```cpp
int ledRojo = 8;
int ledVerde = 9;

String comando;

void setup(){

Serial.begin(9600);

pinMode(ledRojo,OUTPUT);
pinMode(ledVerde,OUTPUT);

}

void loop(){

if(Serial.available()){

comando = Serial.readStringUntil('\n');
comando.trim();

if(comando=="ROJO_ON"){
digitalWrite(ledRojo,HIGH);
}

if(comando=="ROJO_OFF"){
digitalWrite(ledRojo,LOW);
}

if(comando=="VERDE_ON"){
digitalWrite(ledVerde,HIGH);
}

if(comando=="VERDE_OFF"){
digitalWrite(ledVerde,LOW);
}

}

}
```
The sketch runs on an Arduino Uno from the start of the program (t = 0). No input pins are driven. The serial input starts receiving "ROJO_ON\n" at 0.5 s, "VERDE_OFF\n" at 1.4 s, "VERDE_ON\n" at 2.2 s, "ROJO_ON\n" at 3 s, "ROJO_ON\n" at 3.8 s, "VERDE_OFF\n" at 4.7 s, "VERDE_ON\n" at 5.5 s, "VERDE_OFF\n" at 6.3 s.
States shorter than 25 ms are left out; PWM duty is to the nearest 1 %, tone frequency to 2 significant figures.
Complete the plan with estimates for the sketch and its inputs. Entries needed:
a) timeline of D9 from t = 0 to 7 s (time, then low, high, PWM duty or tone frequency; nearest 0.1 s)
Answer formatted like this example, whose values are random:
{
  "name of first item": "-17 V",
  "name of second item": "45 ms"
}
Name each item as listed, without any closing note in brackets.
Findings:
{
  "timeline of D9 from t = 0 to 7 s": "0 s low; 2.2 s high; 4.7 s low; 5.5 s high; 6.3 s low"
}
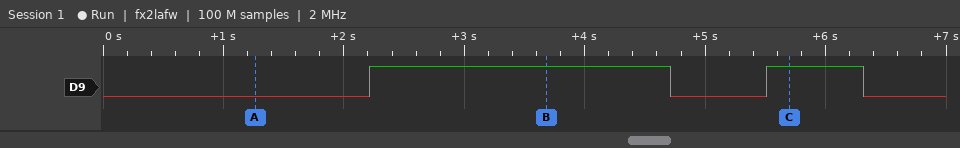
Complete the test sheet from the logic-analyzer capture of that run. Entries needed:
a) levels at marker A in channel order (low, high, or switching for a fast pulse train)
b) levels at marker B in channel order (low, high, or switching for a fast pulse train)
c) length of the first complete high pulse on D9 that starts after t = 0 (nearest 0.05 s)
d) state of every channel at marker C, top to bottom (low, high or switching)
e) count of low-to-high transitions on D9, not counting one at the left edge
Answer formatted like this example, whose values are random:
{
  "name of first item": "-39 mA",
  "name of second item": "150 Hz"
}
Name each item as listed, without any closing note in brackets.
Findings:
{
  "levels at marker A in channel order": "D9 low",
  "levels at marker B in channel order": "D9 high",
  "length of the first complete high pulse on D9 that starts after t = 0": "2.50 s",
  "state of every channel at marker C, top to bottom": "D9 high",
  "count of low-to-high transitions on D9, not counting one at the left edge": "2"
}
